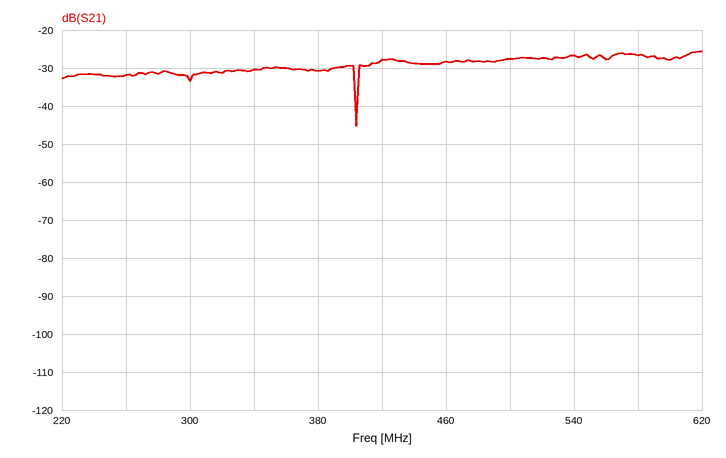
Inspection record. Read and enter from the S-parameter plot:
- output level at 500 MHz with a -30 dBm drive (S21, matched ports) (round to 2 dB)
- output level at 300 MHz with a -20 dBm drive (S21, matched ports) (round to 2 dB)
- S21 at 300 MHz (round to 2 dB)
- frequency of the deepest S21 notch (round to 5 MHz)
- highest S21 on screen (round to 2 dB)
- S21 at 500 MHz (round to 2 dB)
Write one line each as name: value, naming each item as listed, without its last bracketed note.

output level at 500 MHz with a -30 dBm drive (S21, matched ports): -58 dBm
output level at 300 MHz with a -20 dBm drive (S21, matched ports): -54 dBm
S21 at 300 MHz: -34 dB
frequency of the deepest S21 notch: 405 MHz
highest S21 on screen: -26 dB
S21 at 500 MHz: -28 dB
